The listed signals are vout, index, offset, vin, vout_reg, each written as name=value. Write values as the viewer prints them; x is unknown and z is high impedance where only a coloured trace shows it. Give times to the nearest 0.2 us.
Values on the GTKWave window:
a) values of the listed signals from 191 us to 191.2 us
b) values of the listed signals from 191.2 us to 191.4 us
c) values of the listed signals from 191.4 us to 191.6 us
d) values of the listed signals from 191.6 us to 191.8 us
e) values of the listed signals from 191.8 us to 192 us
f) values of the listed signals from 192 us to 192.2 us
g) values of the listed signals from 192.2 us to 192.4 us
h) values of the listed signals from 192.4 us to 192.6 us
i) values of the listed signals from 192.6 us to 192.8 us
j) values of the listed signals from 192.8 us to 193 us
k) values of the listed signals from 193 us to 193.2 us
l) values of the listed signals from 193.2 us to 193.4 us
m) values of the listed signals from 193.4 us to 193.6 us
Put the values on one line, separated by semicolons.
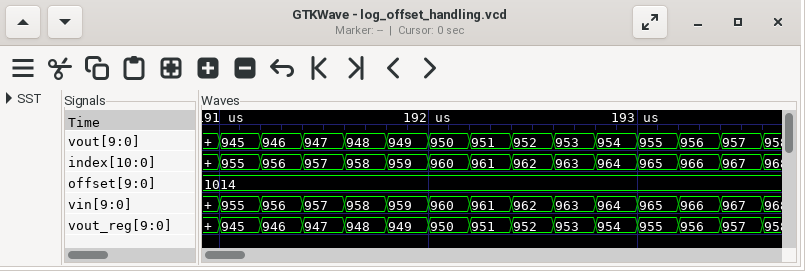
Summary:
vout=945, index=955, offset=1014, vin=955, vout_reg=945; vout=946, index=956, offset=1014, vin=956, vout_reg=946; vout=947, index=957, offset=1014, vin=957, vout_reg=947; vout=948, index=958, offset=1014, vin=958, vout_reg=948; vout=949, index=959, offset=1014, vin=959, vout_reg=949; vout=950, index=960, offset=1014, vin=960, vout_reg=950; vout=951, index=961, offset=1014, vin=961, vout_reg=951; vout=952, index=962, offset=1014, vin=962, vout_reg=952; vout=953, index=963, offset=1014, vin=963, vout_reg=953; vout=954, index=964, offset=1014, vin=964, vout_reg=954; vout=955, index=965, offset=1014, vin=965, vout_reg=955; vout=956, index=966, offset=1014, vin=966, vout_reg=956; vout=957, index=967, offset=1014, vin=967, vout_reg=957
